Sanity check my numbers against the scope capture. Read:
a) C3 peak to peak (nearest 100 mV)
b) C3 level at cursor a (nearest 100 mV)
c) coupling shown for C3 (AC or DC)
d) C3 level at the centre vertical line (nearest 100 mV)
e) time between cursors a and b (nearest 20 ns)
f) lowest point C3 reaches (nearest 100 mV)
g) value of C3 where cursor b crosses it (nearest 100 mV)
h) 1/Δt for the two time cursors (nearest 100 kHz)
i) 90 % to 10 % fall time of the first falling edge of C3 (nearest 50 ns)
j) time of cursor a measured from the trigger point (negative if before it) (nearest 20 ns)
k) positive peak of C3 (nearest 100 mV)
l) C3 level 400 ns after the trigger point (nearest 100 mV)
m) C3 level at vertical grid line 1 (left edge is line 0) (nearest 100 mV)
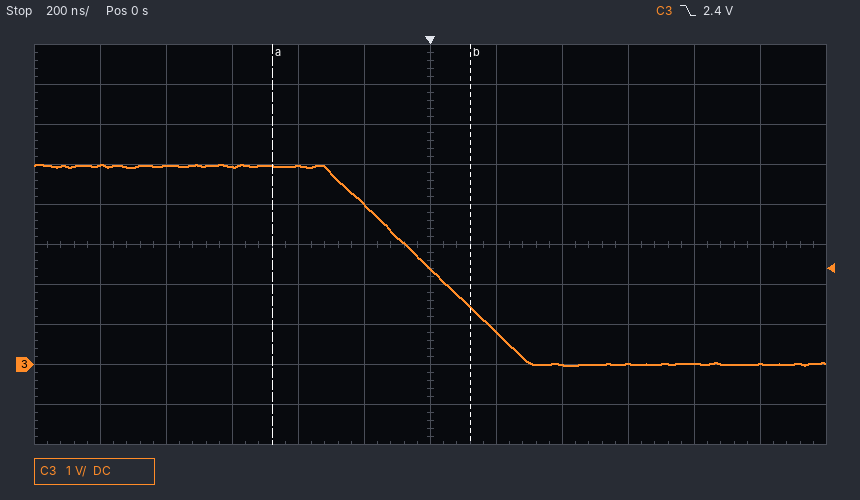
5.0 V
5.0 V
DC
2.4 V
600 ns
0.0 V
1.4 V
1.7 MHz
500 ns
-480 ns
5.0 V
0.0 V
5.0 V
